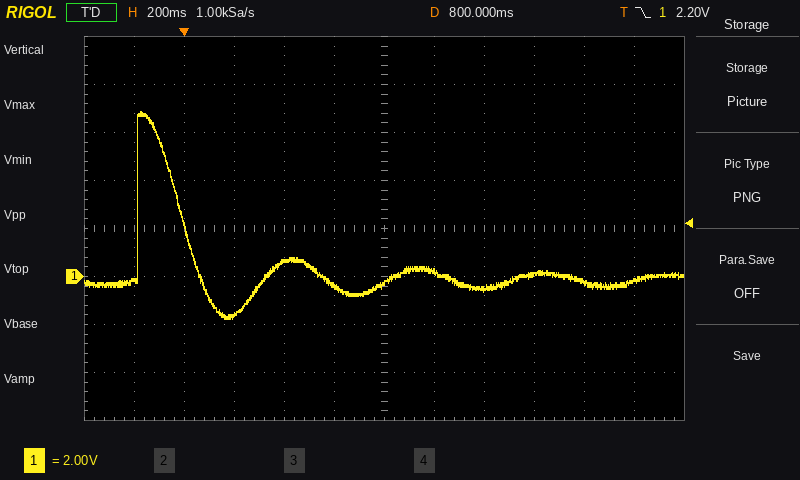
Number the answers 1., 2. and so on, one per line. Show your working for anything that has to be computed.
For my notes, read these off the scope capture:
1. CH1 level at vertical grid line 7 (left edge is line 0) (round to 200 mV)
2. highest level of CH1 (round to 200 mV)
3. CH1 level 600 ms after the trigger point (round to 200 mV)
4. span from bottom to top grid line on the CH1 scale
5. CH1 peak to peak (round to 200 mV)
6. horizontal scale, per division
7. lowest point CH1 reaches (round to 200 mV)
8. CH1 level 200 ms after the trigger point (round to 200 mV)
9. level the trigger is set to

1. 200 mV
2. 6.8 V
3. -400 mV
4. 16 V
5. 6.8 V − (-1.8 V) = 8.6 V
6. 200 ms
7. -1.8 V
8. -1.6 V
9. 2.20 V
